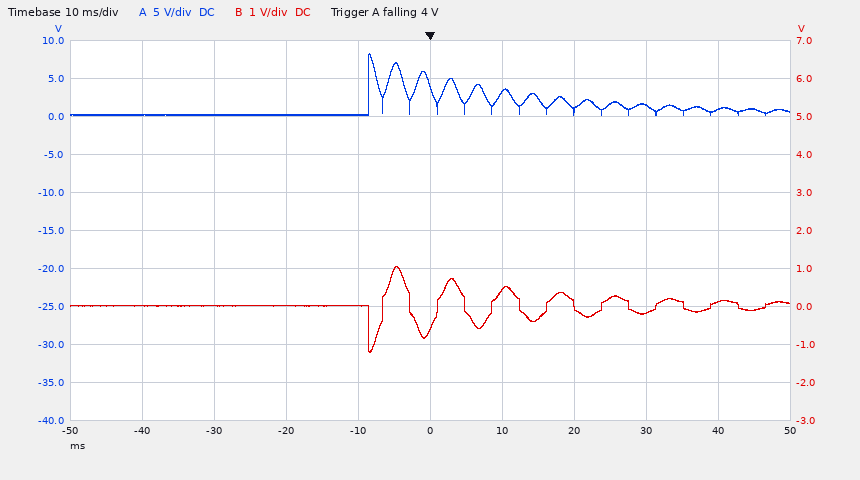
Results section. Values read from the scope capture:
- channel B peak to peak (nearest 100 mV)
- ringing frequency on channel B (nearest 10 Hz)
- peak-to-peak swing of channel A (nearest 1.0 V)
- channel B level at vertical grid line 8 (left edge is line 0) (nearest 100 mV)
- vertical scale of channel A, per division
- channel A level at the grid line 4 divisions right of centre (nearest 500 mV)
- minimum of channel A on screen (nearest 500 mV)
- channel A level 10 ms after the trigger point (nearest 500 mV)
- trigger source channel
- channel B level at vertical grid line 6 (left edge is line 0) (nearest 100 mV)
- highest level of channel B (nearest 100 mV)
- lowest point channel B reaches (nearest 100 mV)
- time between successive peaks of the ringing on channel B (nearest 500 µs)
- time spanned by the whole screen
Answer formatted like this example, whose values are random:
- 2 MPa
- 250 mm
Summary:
- 2.3 V
- 130 Hz
- 8.0 V
- -200 mV
- 5 V
- 1.0 V
- 0.0 V
- 3.0 V
- channel A
- 400 mV
- 1.1 V
- -1.2 V
- 7.5 ms
- 100 ms
